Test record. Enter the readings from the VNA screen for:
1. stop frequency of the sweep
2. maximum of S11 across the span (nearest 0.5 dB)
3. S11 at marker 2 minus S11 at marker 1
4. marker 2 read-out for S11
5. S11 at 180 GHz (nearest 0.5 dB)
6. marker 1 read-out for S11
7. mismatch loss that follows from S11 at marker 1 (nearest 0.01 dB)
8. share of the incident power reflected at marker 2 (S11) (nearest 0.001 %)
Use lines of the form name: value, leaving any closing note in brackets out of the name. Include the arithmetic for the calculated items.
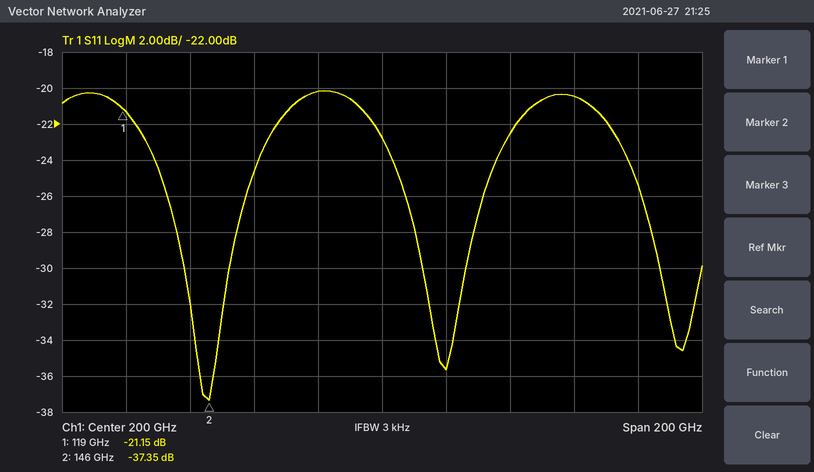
stop frequency of the sweep: 300 GHz
maximum of S11 across the span: -20.0 dB
S11 at marker 2 minus S11 at marker 1: -37.35 − (-21.15) = -16.20 dB
marker 2 read-out for S11: -37.35 dB
S11 at 180 GHz: -20.0 dB
marker 1 read-out for S11: -21.15 dB
mismatch loss that follows from S11 at marker 1: −10 log10(1 − 10^(-21.15/10)) ≈ 0.03 dB
share of the incident power reflected at marker 2 (S11): 10^(-37.35/10) ≈ 0.018 %
